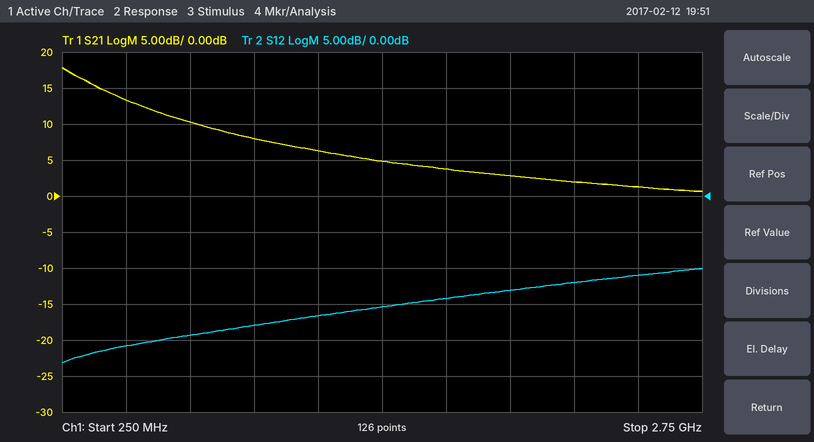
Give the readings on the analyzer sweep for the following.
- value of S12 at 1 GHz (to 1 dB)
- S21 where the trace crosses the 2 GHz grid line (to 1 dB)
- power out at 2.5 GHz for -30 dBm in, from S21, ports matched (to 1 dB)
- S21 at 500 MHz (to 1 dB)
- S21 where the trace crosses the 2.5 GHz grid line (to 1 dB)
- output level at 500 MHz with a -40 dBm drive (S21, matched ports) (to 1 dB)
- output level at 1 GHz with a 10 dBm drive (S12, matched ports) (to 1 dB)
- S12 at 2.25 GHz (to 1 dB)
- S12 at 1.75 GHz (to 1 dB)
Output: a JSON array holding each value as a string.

["-18 dB", "3 dB", "-29 dBm", "13 dB", "1 dB", "-27 dBm", "-8 dBm", "-12 dB", "-14 dB"]
